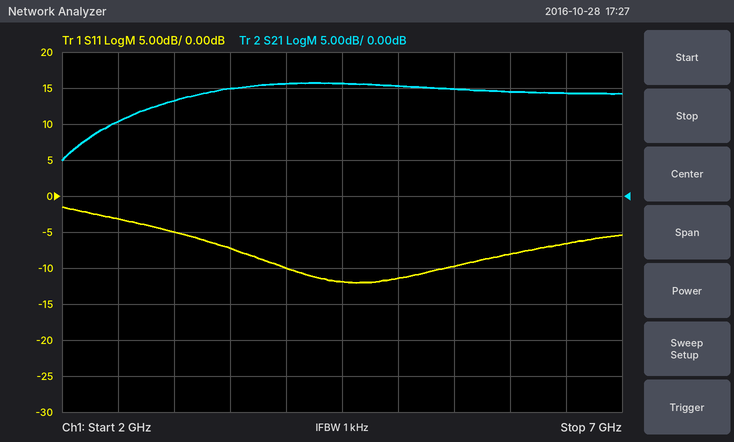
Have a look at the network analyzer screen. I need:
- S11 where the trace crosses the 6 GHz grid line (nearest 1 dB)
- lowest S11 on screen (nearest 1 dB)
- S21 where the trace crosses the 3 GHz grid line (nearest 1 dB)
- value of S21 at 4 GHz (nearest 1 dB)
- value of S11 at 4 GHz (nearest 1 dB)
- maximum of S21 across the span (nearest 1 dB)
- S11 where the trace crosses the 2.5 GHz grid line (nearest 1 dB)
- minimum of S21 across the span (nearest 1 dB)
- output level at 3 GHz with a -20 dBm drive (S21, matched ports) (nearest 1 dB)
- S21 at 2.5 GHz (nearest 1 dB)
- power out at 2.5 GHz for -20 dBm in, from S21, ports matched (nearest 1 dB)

-8 dB
-12 dB
13 dB
16 dB
-10 dB
16 dB
-3 dB
5 dB
-7 dBm
10 dB
-10 dBm
